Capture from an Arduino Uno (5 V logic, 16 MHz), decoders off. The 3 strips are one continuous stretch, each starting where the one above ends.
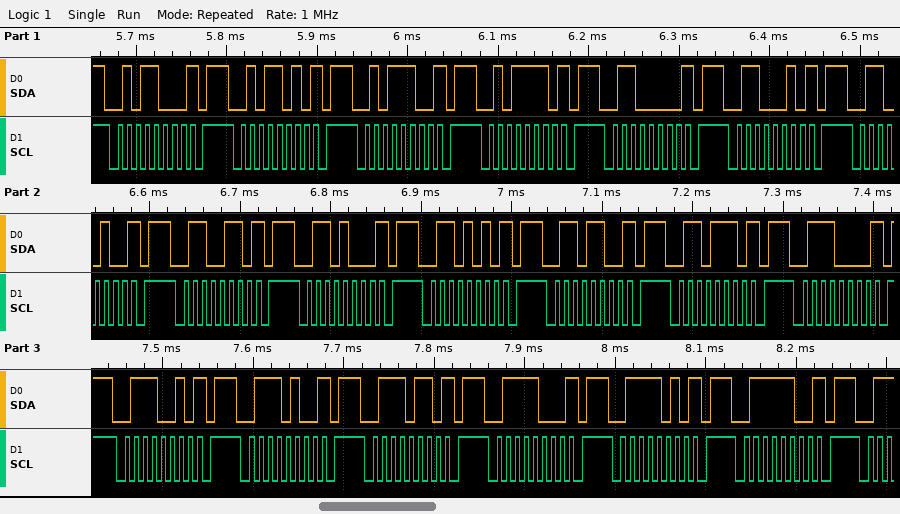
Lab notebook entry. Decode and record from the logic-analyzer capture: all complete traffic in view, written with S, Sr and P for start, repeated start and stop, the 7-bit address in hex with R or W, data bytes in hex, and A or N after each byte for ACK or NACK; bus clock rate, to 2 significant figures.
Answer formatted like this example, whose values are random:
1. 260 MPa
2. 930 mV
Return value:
1. S 2CW N P S 2DW N P S 2EW N P S 2FW N P S 30W N P S 31W N P S 32W N P S 33W N P S 34W N P S 35W N P S 36W N P S 37W N P S 38W N P S 39W N P S 3AW N P S 3BW N P S 3CW N P S 3DW N P S 3EW N P
2. 100 kHz
